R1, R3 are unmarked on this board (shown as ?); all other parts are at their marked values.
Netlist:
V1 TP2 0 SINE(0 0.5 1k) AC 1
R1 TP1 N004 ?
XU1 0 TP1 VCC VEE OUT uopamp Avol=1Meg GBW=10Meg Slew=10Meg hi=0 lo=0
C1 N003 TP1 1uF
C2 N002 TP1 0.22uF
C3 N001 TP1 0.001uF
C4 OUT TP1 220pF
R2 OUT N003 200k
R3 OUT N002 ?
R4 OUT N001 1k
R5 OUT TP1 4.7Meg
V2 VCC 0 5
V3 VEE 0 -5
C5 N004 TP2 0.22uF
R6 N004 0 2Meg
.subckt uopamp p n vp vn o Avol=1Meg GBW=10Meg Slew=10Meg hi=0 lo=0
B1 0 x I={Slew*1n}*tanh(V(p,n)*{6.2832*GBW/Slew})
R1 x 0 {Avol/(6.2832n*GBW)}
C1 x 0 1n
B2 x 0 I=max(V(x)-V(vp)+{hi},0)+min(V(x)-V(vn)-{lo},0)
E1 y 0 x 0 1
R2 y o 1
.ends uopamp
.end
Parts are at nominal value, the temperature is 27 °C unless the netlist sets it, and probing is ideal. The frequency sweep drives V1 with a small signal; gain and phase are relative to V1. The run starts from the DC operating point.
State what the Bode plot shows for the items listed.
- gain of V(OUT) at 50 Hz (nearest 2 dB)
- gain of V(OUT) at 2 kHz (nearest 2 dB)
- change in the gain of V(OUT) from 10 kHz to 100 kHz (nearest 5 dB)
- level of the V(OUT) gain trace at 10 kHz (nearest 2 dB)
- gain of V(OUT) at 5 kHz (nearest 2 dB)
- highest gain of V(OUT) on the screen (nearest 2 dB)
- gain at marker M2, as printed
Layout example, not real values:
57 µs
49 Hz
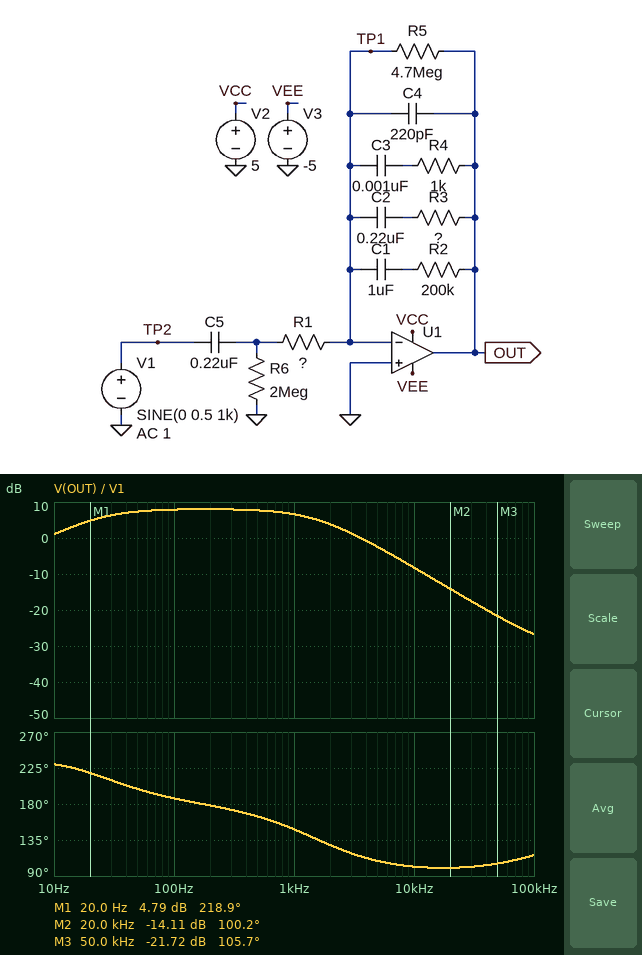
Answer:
8 dB
4 dB
-20 dB
-8 dB
-2 dB
8 dB
-14.11 dB
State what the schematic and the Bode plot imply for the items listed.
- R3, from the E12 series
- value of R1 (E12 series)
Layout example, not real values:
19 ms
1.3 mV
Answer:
150 kΩ
33 kΩ
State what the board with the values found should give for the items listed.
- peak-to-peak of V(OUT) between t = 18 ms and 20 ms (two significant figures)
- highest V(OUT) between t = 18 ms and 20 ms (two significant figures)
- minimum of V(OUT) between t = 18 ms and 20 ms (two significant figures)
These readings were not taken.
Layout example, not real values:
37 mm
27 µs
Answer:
2.1 V
1.1 V
-1.1 V
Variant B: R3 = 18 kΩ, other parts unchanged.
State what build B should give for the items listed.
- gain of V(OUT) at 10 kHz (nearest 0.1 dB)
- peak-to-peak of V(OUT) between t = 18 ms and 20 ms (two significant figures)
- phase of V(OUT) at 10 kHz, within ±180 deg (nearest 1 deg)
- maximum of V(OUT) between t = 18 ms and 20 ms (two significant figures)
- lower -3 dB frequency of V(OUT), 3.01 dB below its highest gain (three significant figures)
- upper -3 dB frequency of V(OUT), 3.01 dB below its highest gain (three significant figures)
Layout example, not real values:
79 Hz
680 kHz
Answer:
-10.4 dB
490 mV
130 deg
250 mV
3.12 Hz
64.0 Hz
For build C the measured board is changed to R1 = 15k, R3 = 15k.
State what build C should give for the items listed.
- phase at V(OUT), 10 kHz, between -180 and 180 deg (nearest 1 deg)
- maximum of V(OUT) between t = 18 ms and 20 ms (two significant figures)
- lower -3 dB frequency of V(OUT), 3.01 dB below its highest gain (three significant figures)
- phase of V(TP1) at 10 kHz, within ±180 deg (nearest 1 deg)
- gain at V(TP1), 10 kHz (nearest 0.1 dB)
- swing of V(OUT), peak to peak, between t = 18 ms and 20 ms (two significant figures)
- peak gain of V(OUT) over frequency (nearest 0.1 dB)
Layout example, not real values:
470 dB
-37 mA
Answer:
135 deg
460 mV
4.10 Hz
45 deg
-64.2 dB
920 mV
-0.7 dB
